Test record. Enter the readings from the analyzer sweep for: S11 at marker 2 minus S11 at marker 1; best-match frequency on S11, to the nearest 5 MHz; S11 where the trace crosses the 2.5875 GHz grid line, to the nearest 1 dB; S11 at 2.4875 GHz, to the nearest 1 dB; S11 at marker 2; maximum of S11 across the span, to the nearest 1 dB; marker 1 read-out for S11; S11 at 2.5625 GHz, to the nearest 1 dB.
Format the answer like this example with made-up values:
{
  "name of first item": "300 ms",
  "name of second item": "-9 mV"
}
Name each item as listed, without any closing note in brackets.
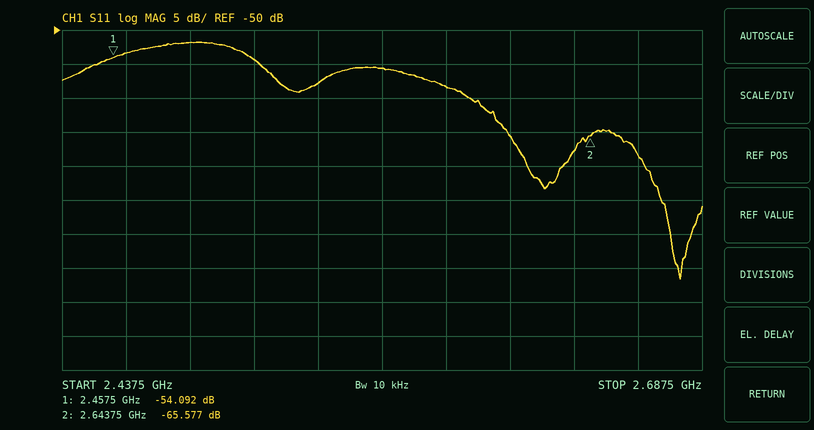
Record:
{
  "S11 at marker 2 minus S11 at marker 1": "-11.485 dB",
  "best-match frequency on S11, to the nearest 5 MHz": "2.680 GHz",
  "S11 where the trace crosses the 2.5875 GHz grid line, to the nearest 1 dB": "-58 dB",
  "S11 at 2.4875 GHz, to the nearest 1 dB": "-52 dB",
  "S11 at marker 2": "-65.577 dB",
  "maximum of S11 across the span, to the nearest 1 dB": "-52 dB",
  "marker 1 read-out for S11": "-54.092 dB",
  "S11 at 2.5625 GHz, to the nearest 1 dB": "-56 dB"
}
